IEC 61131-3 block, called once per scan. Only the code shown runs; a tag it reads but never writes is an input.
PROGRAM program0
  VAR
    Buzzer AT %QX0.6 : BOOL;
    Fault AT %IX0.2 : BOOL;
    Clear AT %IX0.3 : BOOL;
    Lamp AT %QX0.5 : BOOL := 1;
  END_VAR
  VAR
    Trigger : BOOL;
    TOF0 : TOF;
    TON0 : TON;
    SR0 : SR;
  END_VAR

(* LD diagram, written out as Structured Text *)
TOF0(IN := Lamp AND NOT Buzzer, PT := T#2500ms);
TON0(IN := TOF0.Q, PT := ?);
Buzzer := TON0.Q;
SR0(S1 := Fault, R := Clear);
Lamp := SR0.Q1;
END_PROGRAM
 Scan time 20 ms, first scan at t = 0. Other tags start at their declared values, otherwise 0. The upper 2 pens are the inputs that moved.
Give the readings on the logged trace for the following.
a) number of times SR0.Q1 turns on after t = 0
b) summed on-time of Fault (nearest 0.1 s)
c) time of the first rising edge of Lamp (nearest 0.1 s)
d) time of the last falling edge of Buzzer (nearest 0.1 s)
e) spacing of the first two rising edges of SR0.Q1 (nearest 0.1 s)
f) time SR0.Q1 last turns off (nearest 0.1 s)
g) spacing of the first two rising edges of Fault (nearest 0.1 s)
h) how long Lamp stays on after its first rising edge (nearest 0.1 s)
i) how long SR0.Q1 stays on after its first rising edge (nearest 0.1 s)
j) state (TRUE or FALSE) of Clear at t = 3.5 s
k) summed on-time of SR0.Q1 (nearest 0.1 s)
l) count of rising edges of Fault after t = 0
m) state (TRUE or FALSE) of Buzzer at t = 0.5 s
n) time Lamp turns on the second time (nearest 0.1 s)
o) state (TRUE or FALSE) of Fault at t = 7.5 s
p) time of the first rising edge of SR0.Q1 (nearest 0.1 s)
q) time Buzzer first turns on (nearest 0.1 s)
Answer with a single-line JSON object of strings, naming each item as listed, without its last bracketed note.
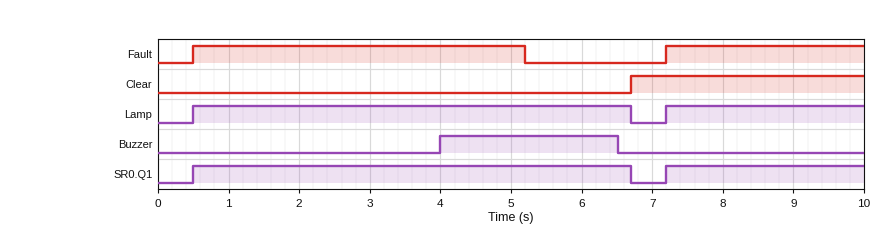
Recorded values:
{"number of times SR0.Q1 turns on after t = 0": "2", "summed on-time of Fault": "7.5 s", "time of the first rising edge of Lamp": "0.5 s", "time of the last falling edge of Buzzer": "6.5 s", "spacing of the first two rising edges of SR0.Q1": "6.7 s", "time SR0.Q1 last turns off": "6.7 s", "spacing of the first two rising edges of Fault": "6.7 s", "how long Lamp stays on after its first rising edge": "6.2 s", "how long SR0.Q1 stays on after its first rising edge": "6.2 s", "state (TRUE or FALSE) of Clear at t = 3.5 s": "FALSE", "summed on-time of SR0.Q1": "9.0 s", "count of rising edges of Fault after t = 0": "2", "state (TRUE or FALSE) of Buzzer at t = 0.5 s": "FALSE", "time Lamp turns on the second time": "7.2 s", "state (TRUE or FALSE) of Fault at t = 7.5 s": "TRUE", "time of the first rising edge of SR0.Q1": "0.5 s", "time Buzzer first turns on": "4.0 s"}
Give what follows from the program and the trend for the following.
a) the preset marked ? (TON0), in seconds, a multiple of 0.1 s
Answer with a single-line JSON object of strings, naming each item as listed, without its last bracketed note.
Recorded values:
{"the preset marked ? (TON0), in seconds, a multiple of 0.1 s": "4.0 s"}
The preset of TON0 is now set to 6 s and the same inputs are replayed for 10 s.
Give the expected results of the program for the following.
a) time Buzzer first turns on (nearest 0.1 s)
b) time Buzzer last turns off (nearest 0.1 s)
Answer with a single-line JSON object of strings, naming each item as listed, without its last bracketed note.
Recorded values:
{"time Buzzer first turns on": "6.0 s", "time Buzzer last turns off": "8.5 s"}
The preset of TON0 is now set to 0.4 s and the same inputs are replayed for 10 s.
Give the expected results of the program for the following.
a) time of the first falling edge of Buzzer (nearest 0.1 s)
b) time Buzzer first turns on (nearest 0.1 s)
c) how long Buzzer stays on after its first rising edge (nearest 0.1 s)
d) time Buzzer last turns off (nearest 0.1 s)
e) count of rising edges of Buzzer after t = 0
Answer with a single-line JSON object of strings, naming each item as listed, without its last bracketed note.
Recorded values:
{"time of the first falling edge of Buzzer": "2.5 s", "time Buzzer first turns on": "0.4 s", "how long Buzzer stays on after its first rising edge": "2.1 s", "time Buzzer last turns off": "8.4 s", "count of rising edges of Buzzer after t = 0": "4"}
